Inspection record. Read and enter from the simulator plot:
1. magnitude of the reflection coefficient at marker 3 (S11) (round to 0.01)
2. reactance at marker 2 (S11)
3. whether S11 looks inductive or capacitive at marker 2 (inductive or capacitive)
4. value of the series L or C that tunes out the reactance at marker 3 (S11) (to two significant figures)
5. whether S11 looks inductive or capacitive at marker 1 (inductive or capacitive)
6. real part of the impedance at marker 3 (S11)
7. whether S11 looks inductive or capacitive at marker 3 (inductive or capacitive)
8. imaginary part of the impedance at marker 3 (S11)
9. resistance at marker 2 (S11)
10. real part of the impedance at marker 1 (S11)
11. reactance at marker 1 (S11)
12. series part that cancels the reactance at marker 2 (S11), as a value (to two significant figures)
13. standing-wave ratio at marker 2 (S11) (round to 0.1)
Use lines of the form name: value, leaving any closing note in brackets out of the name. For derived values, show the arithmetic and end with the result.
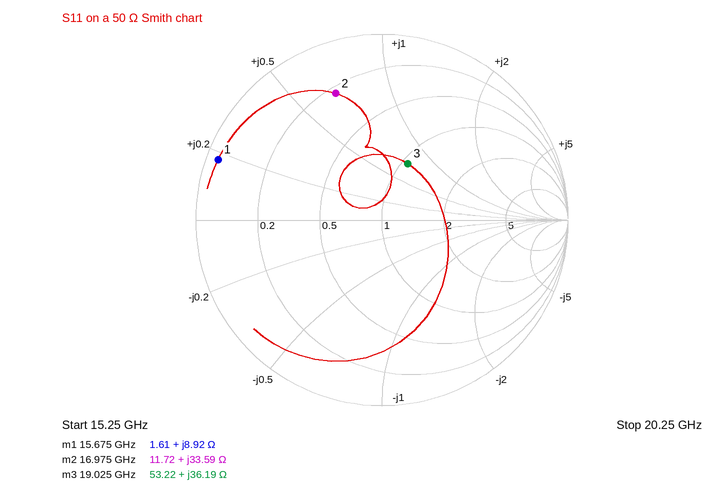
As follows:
magnitude of the reflection coefficient at marker 3 (S11): 0.33
reactance at marker 2: +33.59 Ω
whether S11 looks inductive or capacitive at marker 2: inductive
value of the series L or C that tunes out the reactance at marker 3 (S11): C = 1/(2π × 19.025 GHz × 36.19 Ω) ≈ 231 fF, so 230 fF to two significant figures
whether S11 looks inductive or capacitive at marker 1: inductive
real part of the impedance at marker 3: 53.22 Ω
whether S11 looks inductive or capacitive at marker 3: inductive
imaginary part of the impedance at marker 3: +36.19 Ω
resistance at marker 2: 11.72 Ω
real part of the impedance at marker 1: 1.61 Ω
reactance at marker 1: +8.92 Ω
series part that cancels the reactance at marker 2 (S11), as a value: C = 1/(2π × 16.975 GHz × 33.59 Ω) ≈ 279 fF, so 280 fF to two significant figures
standing-wave ratio at marker 2 (S11): 6.3
